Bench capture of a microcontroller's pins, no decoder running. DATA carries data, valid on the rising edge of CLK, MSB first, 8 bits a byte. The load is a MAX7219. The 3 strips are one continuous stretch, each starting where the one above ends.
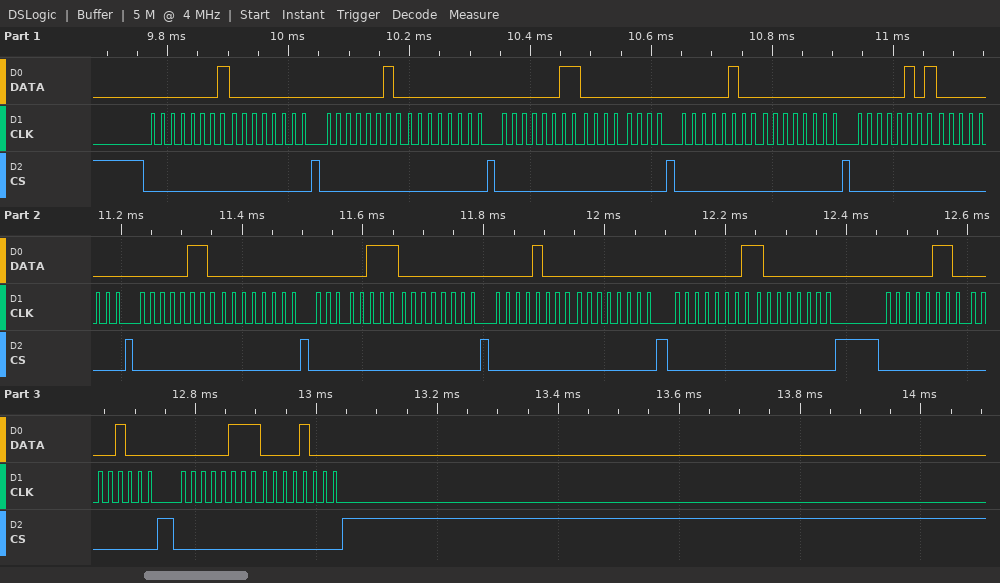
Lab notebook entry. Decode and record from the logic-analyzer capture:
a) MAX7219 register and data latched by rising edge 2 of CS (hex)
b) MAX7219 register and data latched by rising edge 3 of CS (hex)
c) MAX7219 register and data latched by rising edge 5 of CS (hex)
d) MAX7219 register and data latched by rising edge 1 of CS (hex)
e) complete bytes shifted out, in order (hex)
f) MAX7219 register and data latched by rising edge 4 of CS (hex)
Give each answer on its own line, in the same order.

register 0x2, data 0x00
register 0x3, data 0x00
register 0x5, data 0x00
register 0x1, data 0x00
01 00 02 00 03 00 04 00 05 00 06 00 07 00 08 00 01 80 06 08 07 08
register 0x4, data 0x00
